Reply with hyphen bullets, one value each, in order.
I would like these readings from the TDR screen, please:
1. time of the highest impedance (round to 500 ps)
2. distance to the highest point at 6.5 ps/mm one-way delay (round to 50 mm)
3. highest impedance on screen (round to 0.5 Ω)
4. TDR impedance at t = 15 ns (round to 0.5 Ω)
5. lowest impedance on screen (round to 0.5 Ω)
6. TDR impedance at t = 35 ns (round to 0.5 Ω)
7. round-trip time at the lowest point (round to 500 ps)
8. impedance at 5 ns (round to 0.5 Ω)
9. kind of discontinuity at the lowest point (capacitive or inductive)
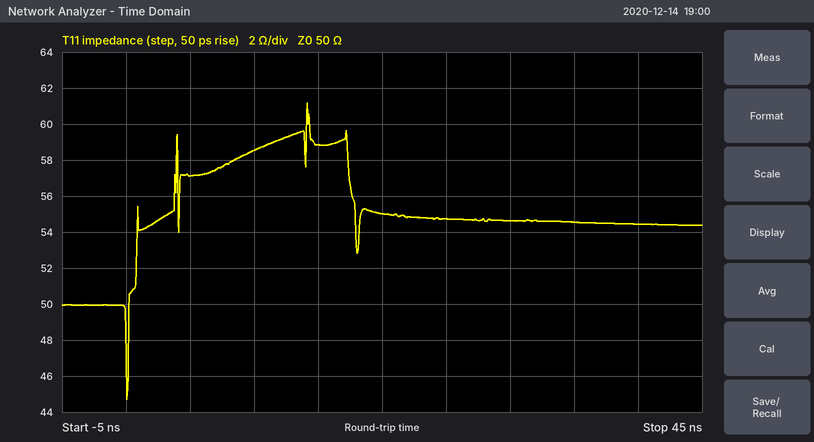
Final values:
- 14.0 ns
- 1.10 m
- 61.0 Ω
- 59.0 Ω
- 44.5 Ω
- 54.5 Ω
- 0.0 ns
- 57.0 Ω
- capacitive
